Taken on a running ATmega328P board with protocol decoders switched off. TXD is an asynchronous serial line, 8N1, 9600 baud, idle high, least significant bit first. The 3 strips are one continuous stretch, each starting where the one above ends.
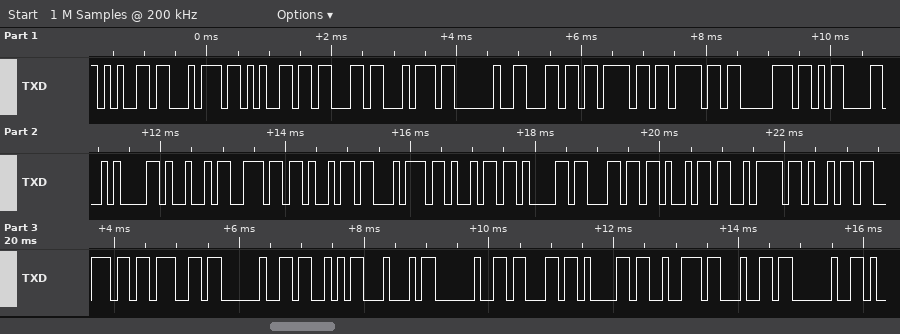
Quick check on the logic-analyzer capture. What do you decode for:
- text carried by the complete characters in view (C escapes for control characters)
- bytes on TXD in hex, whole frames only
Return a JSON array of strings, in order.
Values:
["\"etect loop\\r\\nInitializing SD card \"", "0x65 0x74 0x65 0x63 0x74 0x20 0x6C 0x6F 0x6F 0x70 0x0D 0x0A 0x49 0x6E 0x69 0x74 0x69 0x61 0x6C 0x69 0x7A 0x69 0x6E 0x67 0x20 0x53 0x44 0x20 0x63 0x61 0x72 0x64 0x20"]
